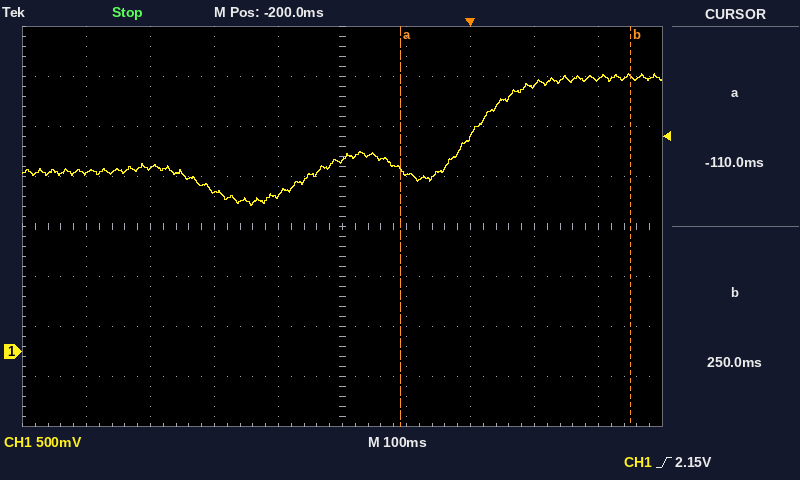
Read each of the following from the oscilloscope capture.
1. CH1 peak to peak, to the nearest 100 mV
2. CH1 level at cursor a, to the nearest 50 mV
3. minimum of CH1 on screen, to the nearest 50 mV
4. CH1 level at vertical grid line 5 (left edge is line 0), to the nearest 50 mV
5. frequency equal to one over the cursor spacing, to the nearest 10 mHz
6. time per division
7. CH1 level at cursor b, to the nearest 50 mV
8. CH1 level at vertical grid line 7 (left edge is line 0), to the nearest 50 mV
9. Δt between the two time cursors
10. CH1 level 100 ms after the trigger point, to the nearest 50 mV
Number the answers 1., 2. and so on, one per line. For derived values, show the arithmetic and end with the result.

1. 1.30 V
2. 1.80 V
3. 1.45 V
4. 1.90 V
5. 1 / 360 ms ≈ 2.78 Hz
6. 100 ms
7. 2.75 V
8. 2.15 V
9. 250 ms − (-110 ms) = 360 ms
10. 2.65 V
